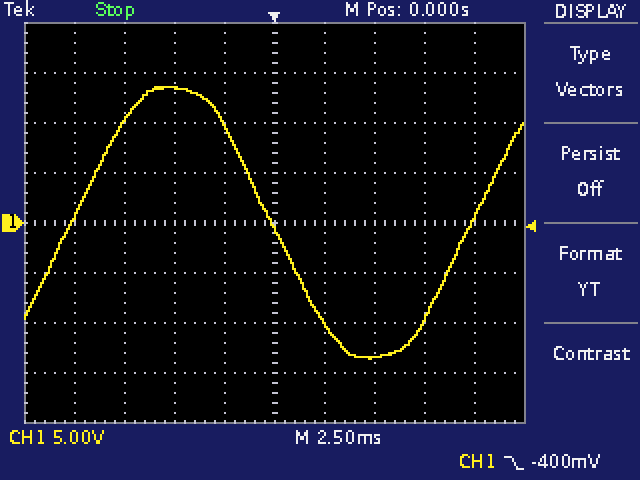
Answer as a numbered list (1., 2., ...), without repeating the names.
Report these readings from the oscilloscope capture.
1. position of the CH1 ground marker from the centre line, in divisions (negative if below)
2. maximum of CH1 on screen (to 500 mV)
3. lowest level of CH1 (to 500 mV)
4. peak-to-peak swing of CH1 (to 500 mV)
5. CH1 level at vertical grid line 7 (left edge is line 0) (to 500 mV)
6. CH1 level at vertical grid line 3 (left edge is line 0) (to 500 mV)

1. 0.0 div
2. 13.5 V
3. -13.5 V
4. 27.0 V
5. -13.5 V
6. 13.5 V
